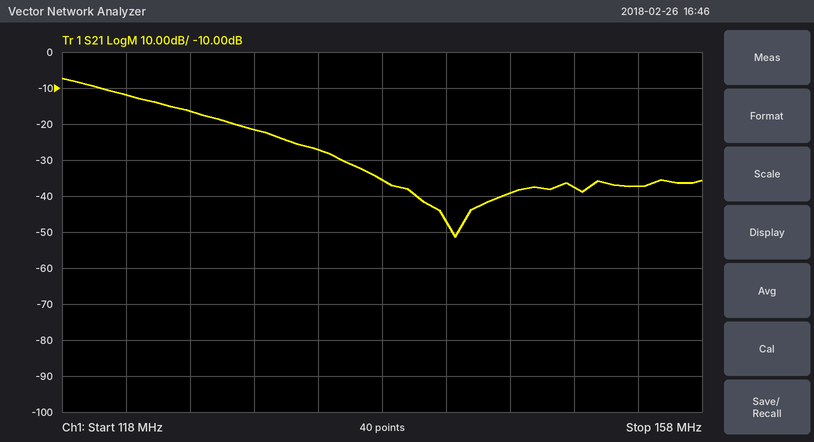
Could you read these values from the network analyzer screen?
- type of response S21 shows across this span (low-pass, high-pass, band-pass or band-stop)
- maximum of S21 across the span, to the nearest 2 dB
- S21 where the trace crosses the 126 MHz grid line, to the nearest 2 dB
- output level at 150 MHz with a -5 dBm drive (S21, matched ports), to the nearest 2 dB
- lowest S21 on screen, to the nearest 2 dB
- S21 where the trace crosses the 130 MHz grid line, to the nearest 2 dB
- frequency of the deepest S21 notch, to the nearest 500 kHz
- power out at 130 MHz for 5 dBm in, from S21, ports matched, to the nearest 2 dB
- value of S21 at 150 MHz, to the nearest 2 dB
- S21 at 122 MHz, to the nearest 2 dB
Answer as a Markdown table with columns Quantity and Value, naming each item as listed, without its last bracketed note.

| Quantity | Value |
|---|---|
| type of response S21 shows across this span | low-pass |
| maximum of S21 across the span, to the nearest 2 dB | -8 dB |
| S21 where the trace crosses the 126 MHz grid line, to the nearest 2 dB | -16 dB |
| output level at 150 MHz with a -5 dBm drive (S21, matched ports), to the nearest 2 dB | -42 dBm |
| lowest S21 on screen, to the nearest 2 dB | -52 dB |
| S21 where the trace crosses the 130 MHz grid line, to the nearest 2 dB | -22 dB |
| frequency of the deepest S21 notch, to the nearest 500 kHz | 142.5 MHz |
| power out at 130 MHz for 5 dBm in, from S21, ports matched, to the nearest 2 dB | -16 dBm |
| value of S21 at 150 MHz, to the nearest 2 dB | -38 dB |
| S21 at 122 MHz, to the nearest 2 dB | -12 dB |
